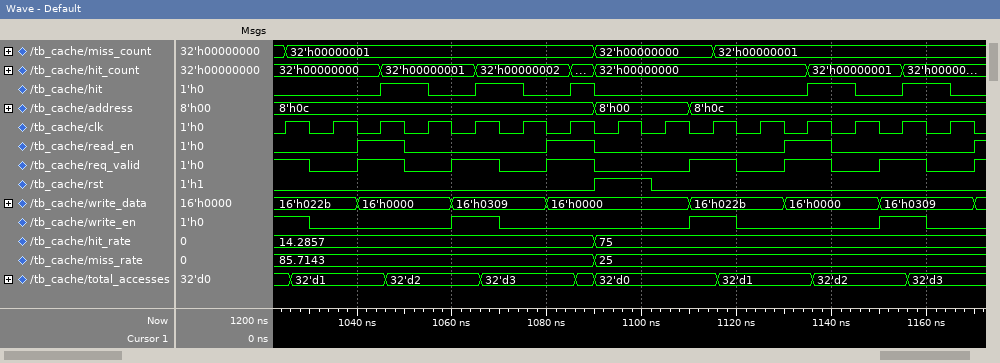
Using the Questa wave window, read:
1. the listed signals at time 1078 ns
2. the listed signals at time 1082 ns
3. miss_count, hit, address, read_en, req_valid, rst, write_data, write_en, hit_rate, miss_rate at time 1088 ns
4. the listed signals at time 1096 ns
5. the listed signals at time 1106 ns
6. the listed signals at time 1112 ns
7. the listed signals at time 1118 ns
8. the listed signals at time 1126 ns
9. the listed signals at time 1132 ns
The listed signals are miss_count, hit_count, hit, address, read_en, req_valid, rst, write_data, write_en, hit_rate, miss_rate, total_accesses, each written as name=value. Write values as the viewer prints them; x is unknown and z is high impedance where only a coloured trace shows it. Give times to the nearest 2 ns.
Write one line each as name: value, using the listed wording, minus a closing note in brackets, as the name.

the listed signals at time 1078 ns: miss_count=32'h00000001, hit_count=32'h00000002, hit=0, address=8'h0c, read_en=0, req_valid=0, rst=0, write_data=16'h0309, write_en=0, hit_rate=14.2857, miss_rate=85.7143, total_accesses=32'd3
the listed signals at time 1082 ns: miss_count=32'h00000001, hit_count=32'h00000002, hit=0, address=8'h0c, read_en=1, req_valid=1, rst=0, write_data=16'h0000, write_en=0, hit_rate=14.2857, miss_rate=85.7143, total_accesses=32'd3
miss_count, hit, address, read_en, req_valid, rst, write_data, write_en, hit_rate, miss_rate at time 1088 ns: miss_count=32'h00000001, hit=1, address=8'h0c, read_en=1, req_valid=1, rst=0, write_data=16'h0000, write_en=0, hit_rate=14.2857, miss_rate=85.7143
the listed signals at time 1096 ns: miss_count=32'h00000000, hit_count=32'h00000000, hit=0, address=8'h00, read_en=0, req_valid=0, rst=1, write_data=16'h0000, write_en=0, hit_rate=75, miss_rate=25, total_accesses=32'd0
the listed signals at time 1106 ns: miss_count=32'h00000000, hit_count=32'h00000000, hit=0, address=8'h00, read_en=0, req_valid=0, rst=0, write_data=16'h0000, write_en=0, hit_rate=75, miss_rate=25, total_accesses=32'd0
the listed signals at time 1112 ns: miss_count=32'h00000000, hit_count=32'h00000000, hit=0, address=8'h0c, read_en=0, req_valid=1, rst=0, write_data=16'h022b, write_en=1, hit_rate=75, miss_rate=25, total_accesses=32'd0
the listed signals at time 1118 ns: miss_count=32'h00000001, hit_count=32'h00000000, hit=0, address=8'h0c, read_en=0, req_valid=1, rst=0, write_data=16'h022b, write_en=1, hit_rate=75, miss_rate=25, total_accesses=32'd1
the listed signals at time 1126 ns: miss_count=32'h00000001, hit_count=32'h00000000, hit=0, address=8'h0c, read_en=0, req_valid=0, rst=0, write_data=16'h022b, write_en=0, hit_rate=75, miss_rate=25, total_accesses=32'd1
the listed signals at time 1132 ns: miss_count=32'h00000001, hit_count=32'h00000000, hit=0, address=8'h0c, read_en=1, req_valid=1, rst=0, write_data=16'h0000, write_en=0, hit_rate=75, miss_rate=25, total_accesses=32'd1
